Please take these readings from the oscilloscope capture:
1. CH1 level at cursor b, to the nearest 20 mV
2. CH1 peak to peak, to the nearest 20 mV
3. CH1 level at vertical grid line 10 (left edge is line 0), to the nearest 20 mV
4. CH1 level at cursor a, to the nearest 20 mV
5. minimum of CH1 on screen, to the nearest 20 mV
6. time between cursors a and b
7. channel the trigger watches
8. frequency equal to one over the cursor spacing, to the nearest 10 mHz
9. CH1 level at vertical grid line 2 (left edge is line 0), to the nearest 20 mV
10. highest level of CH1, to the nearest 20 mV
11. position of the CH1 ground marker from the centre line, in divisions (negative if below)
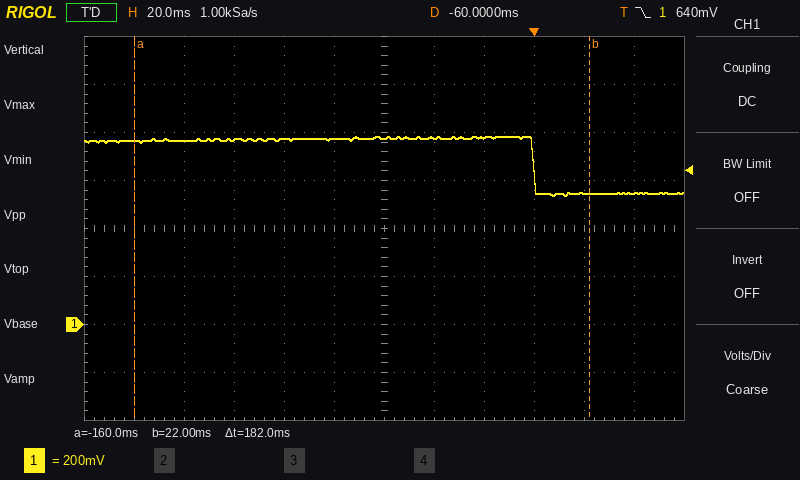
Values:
540 mV
240 mV
540 mV
760 mV
540 mV
182 ms
CH1
5.49 Hz
760 mV
780 mV
-2.0 div
